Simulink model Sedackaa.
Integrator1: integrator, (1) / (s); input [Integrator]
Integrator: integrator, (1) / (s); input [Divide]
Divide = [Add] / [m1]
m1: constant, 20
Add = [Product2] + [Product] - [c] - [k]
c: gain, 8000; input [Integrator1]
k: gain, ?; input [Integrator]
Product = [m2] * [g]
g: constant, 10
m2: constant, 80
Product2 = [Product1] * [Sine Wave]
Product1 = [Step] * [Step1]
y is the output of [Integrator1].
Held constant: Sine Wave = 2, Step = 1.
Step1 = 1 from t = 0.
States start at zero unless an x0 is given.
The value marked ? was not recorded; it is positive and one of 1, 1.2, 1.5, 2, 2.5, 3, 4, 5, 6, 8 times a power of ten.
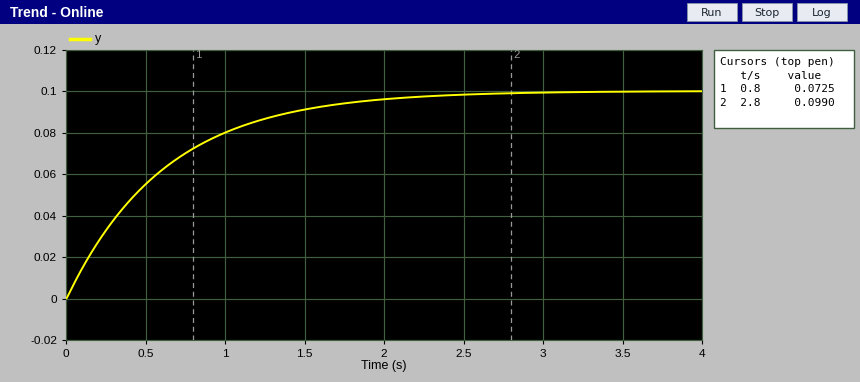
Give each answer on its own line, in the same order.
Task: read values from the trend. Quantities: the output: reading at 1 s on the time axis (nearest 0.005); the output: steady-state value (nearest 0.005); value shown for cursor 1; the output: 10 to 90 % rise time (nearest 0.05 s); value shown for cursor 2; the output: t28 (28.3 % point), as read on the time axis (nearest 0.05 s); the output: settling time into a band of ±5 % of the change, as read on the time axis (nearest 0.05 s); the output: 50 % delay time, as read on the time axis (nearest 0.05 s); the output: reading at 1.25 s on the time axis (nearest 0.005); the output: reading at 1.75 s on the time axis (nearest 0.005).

0.080
0.100
0.0725
1.35 s
0.0990
0.20 s
1.85 s
0.45 s
0.085
0.095
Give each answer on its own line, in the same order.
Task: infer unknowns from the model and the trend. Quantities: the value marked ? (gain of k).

5000
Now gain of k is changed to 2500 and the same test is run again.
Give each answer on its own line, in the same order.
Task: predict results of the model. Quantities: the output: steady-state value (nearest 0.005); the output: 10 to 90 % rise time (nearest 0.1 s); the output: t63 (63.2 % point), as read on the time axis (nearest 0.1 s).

0.100
0.7 s
0.3 s
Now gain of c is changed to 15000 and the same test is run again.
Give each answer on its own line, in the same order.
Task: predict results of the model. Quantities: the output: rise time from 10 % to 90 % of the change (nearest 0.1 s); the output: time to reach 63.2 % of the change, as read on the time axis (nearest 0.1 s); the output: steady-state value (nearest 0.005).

0.7 s
0.3 s
0.055
